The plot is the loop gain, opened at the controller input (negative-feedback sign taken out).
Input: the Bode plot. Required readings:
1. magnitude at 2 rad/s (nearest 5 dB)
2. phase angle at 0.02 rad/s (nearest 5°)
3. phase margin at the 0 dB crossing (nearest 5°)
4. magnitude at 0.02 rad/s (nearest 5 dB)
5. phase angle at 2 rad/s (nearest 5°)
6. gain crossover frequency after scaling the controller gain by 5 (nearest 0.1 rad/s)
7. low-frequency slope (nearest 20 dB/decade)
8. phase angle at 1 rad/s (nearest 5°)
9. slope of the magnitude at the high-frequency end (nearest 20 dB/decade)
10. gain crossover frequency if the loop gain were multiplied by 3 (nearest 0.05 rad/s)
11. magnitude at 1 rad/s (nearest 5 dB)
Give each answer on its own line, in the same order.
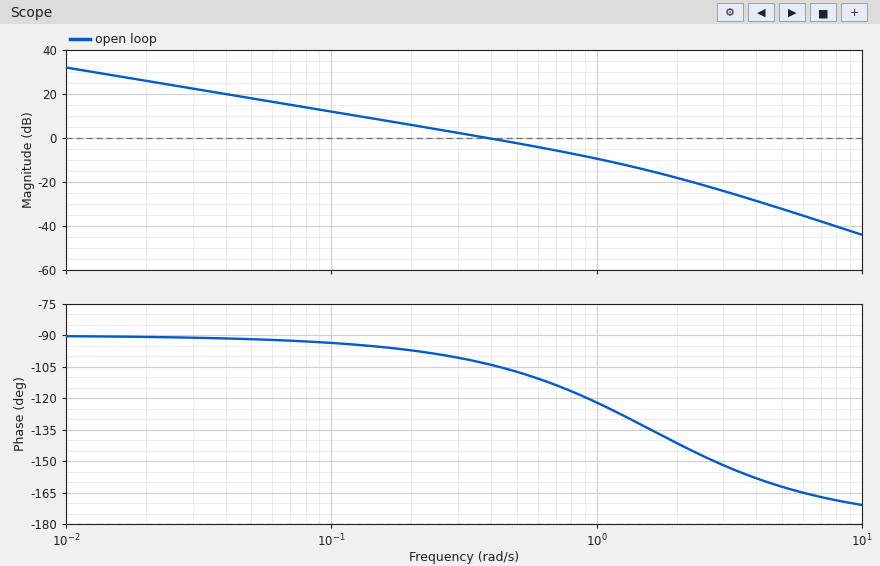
-20 dB
-90°
75°
25 dB
-140°
1.5 rad/s
-20 dB/decade
-120°
-40 dB/decade
1.00 rad/s
-10 dB
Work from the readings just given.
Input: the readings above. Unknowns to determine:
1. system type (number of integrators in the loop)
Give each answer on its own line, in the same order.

1
